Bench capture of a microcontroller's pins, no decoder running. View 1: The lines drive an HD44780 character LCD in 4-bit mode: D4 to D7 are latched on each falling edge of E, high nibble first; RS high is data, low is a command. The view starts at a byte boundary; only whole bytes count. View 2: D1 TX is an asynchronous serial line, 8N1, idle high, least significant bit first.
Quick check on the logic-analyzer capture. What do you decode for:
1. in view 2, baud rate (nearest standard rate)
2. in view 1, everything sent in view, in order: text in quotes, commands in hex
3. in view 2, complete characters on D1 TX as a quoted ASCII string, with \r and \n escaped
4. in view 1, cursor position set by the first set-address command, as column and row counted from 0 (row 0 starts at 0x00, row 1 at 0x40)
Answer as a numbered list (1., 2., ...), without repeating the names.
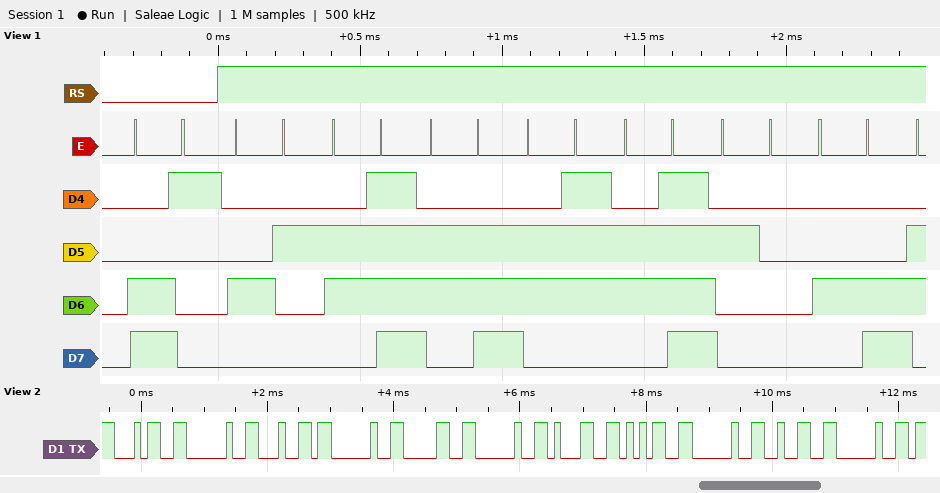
1. 9600 baud
2. 0xC1 "Bongo L"
3. "4 d 0 15 2 "
4. column 1, row 1
